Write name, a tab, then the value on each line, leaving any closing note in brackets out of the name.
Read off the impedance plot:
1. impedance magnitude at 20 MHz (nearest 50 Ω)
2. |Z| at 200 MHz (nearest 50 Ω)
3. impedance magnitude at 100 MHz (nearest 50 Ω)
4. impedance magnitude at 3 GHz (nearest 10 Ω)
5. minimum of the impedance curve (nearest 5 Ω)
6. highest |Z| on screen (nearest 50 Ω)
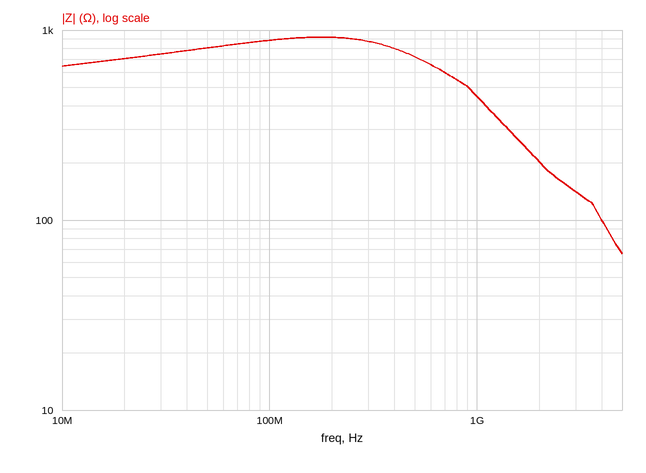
impedance magnitude at 20 MHz	700 Ω
|Z| at 200 MHz	900 Ω
impedance magnitude at 100 MHz	900 Ω
impedance magnitude at 3 GHz	140 Ω
minimum of the impedance curve	65 Ω
highest |Z| on screen	900 Ω
